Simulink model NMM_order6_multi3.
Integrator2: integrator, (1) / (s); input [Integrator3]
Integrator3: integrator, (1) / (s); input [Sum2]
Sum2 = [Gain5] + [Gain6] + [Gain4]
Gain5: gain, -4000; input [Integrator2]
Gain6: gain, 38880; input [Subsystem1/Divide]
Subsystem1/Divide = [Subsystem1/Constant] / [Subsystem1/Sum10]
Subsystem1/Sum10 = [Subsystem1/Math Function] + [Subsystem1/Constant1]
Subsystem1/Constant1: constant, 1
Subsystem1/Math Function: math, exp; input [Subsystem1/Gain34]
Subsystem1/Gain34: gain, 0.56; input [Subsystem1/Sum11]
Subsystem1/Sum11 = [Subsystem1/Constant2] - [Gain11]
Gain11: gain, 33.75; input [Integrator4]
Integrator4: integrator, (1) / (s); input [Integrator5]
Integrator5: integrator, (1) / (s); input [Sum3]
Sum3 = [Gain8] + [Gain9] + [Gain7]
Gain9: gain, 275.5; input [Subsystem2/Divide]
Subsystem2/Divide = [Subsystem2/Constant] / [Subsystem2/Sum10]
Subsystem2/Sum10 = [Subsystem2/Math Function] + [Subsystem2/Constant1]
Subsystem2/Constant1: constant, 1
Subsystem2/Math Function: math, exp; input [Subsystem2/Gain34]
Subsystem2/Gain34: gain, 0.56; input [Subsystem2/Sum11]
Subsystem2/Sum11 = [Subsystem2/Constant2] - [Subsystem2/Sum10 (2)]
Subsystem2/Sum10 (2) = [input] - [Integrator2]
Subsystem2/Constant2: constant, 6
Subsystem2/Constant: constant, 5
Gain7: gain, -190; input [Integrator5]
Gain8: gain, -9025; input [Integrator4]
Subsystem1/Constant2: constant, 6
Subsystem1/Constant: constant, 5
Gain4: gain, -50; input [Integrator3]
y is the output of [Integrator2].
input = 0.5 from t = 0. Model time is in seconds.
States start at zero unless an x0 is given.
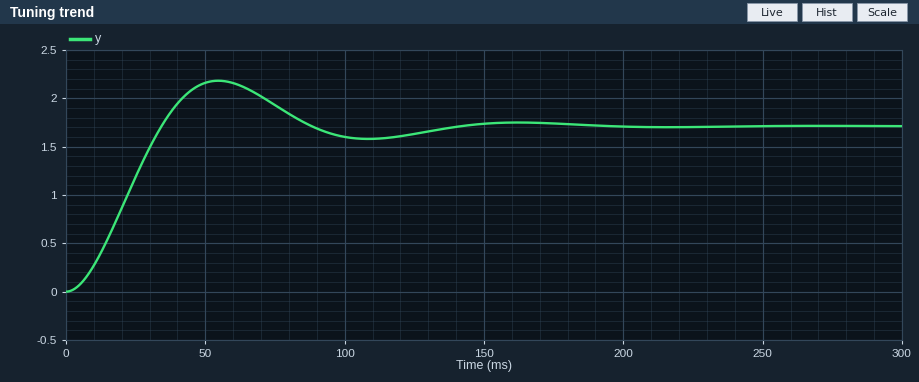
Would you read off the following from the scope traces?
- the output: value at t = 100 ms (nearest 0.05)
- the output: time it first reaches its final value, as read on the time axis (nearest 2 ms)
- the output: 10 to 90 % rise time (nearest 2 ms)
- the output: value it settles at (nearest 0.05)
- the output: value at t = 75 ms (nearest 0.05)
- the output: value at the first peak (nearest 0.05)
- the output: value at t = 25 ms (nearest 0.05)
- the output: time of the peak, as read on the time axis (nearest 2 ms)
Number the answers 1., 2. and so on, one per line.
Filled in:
1. 1.60
2. 34 ms
3. 24 ms
4. 1.70
5. 1.95
6. 2.20
7. 1.20
8. 54 ms
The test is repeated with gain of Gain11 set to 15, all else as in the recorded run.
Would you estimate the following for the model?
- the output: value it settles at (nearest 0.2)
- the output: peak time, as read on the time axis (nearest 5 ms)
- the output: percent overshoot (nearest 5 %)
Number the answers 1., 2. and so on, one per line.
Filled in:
1. 1.6
2. 55 ms
3. 25 %
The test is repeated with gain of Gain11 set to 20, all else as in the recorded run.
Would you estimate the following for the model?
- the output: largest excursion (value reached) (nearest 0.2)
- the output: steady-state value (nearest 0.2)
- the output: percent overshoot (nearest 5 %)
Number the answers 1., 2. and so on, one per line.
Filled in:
1. 2.2
2. 1.6
3. 25 %
